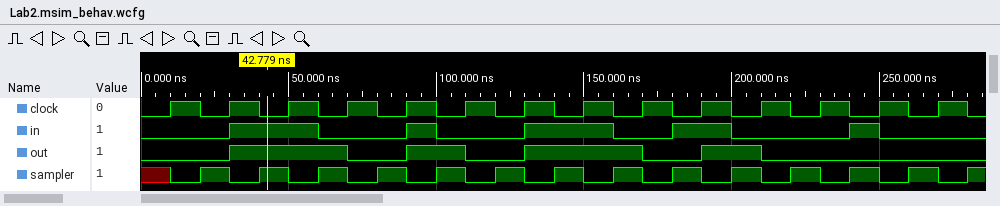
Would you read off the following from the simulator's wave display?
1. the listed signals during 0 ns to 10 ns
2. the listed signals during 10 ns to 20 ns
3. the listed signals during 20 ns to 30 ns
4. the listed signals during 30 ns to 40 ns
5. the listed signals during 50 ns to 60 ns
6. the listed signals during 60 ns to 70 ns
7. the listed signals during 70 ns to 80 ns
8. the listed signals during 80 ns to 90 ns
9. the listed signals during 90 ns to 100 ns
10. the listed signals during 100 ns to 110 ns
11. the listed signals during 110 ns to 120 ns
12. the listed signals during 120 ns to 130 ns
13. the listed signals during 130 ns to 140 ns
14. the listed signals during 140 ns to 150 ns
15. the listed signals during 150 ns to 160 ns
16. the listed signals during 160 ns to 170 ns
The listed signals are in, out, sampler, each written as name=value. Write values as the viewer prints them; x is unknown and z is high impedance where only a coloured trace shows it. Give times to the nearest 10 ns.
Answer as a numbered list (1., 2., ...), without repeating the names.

1. in=0, out=0, sampler=x
2. in=0, out=0, sampler=0
3. in=0, out=0, sampler=1
4. in=1, out=1, sampler=0
5. in=1, out=1, sampler=0
6. in=0, out=1, sampler=1
7. in=0, out=0, sampler=0
8. in=0, out=0, sampler=1
9. in=1, out=1, sampler=0
10. in=0, out=1, sampler=1
11. in=0, out=0, sampler=0
12. in=0, out=0, sampler=1
13. in=1, out=1, sampler=0
14. in=1, out=1, sampler=1
15. in=1, out=1, sampler=0
16. in=0, out=1, sampler=1
